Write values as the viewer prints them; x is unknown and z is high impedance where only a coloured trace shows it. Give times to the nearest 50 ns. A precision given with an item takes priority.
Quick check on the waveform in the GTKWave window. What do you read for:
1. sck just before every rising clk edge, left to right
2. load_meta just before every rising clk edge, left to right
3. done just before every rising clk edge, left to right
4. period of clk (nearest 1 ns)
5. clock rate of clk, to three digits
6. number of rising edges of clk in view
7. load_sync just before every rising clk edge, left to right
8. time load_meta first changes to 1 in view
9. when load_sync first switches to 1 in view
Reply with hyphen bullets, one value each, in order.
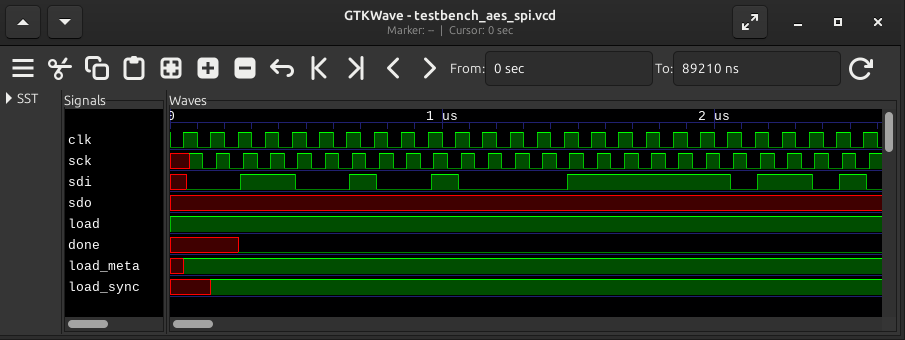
- x 0 0 0 0 0 0 0 0 0 0 0 0 0 0 0 0 0 0 0 0 0 0 0 0 0
- x 1 1 1 1 1 1 1 1 1 1 1 1 1 1 1 1 1 1 1 1 1 1 1 1 1
- x x x 0 0 0 0 0 0 0 0 0 0 0 0 0 0 0 0 0 0 0 0 0 0 0
- 100 ns
- 10.0 MHz
- 26
- x x 1 1 1 1 1 1 1 1 1 1 1 1 1 1 1 1 1 1 1 1 1 1 1 1
- 50 ns
- 150 ns
